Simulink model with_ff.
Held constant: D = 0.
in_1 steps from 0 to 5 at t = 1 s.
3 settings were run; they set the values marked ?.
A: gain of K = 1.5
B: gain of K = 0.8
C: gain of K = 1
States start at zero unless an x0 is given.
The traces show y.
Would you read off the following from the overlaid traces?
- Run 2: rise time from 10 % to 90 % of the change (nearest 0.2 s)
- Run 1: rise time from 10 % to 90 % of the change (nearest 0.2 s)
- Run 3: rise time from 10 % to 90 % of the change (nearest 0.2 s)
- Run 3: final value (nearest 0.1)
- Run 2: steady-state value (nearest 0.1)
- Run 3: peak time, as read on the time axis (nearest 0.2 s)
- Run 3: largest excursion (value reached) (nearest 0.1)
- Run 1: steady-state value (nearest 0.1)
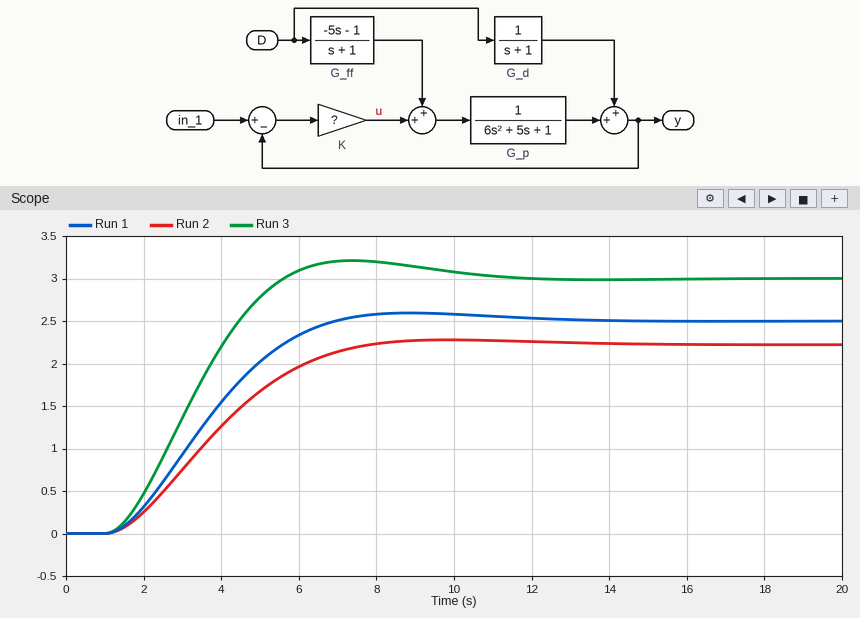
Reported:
4.2 s
3.8 s
3.0 s
3.0
2.2
7.4 s
3.2
2.5
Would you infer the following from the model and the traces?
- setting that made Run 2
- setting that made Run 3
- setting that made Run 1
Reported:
B
A
C
